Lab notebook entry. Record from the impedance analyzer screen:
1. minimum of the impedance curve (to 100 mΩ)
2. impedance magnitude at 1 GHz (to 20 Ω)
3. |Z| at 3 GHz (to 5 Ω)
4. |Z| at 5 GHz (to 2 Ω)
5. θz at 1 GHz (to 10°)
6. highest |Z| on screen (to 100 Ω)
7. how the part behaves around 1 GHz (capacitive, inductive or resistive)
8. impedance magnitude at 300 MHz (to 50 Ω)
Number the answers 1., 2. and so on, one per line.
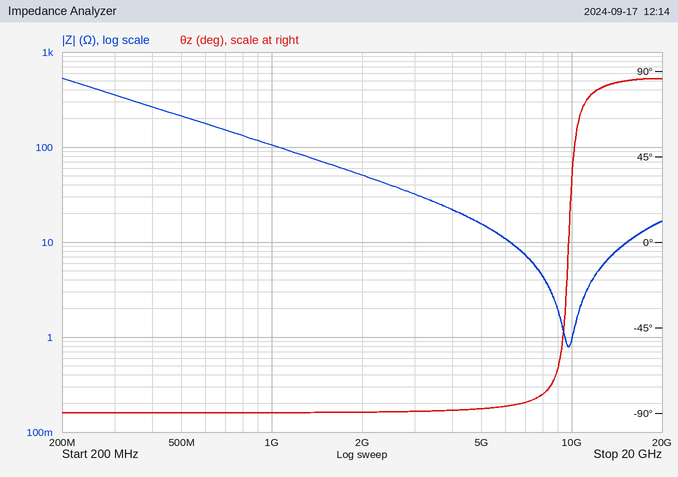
1. 800 mΩ
2. 100 Ω
3. 30 Ω
4. 16 Ω
5. -90°
6. 500 Ω
7. capacitive
8. 350 Ω
